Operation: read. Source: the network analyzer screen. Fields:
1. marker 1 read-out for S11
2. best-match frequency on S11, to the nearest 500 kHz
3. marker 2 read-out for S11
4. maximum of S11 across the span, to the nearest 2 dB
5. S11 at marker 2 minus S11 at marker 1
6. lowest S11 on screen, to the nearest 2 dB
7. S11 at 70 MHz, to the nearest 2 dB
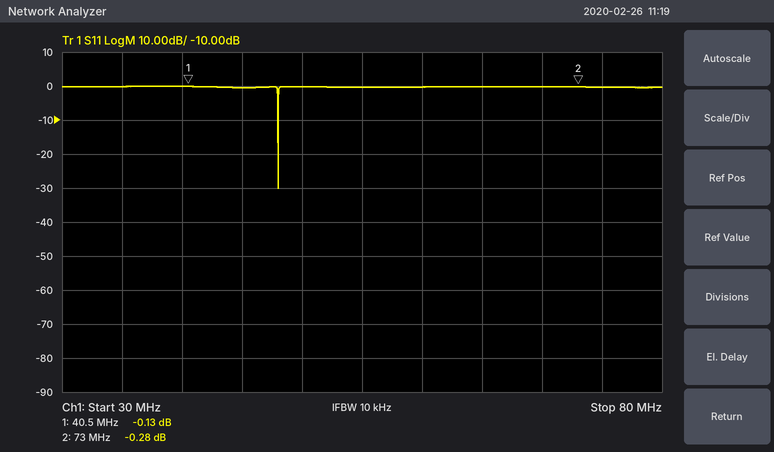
-0.13 dB
48.0 MHz
-0.28 dB
0 dB
-0.15 dB
-30 dB
0 dB
